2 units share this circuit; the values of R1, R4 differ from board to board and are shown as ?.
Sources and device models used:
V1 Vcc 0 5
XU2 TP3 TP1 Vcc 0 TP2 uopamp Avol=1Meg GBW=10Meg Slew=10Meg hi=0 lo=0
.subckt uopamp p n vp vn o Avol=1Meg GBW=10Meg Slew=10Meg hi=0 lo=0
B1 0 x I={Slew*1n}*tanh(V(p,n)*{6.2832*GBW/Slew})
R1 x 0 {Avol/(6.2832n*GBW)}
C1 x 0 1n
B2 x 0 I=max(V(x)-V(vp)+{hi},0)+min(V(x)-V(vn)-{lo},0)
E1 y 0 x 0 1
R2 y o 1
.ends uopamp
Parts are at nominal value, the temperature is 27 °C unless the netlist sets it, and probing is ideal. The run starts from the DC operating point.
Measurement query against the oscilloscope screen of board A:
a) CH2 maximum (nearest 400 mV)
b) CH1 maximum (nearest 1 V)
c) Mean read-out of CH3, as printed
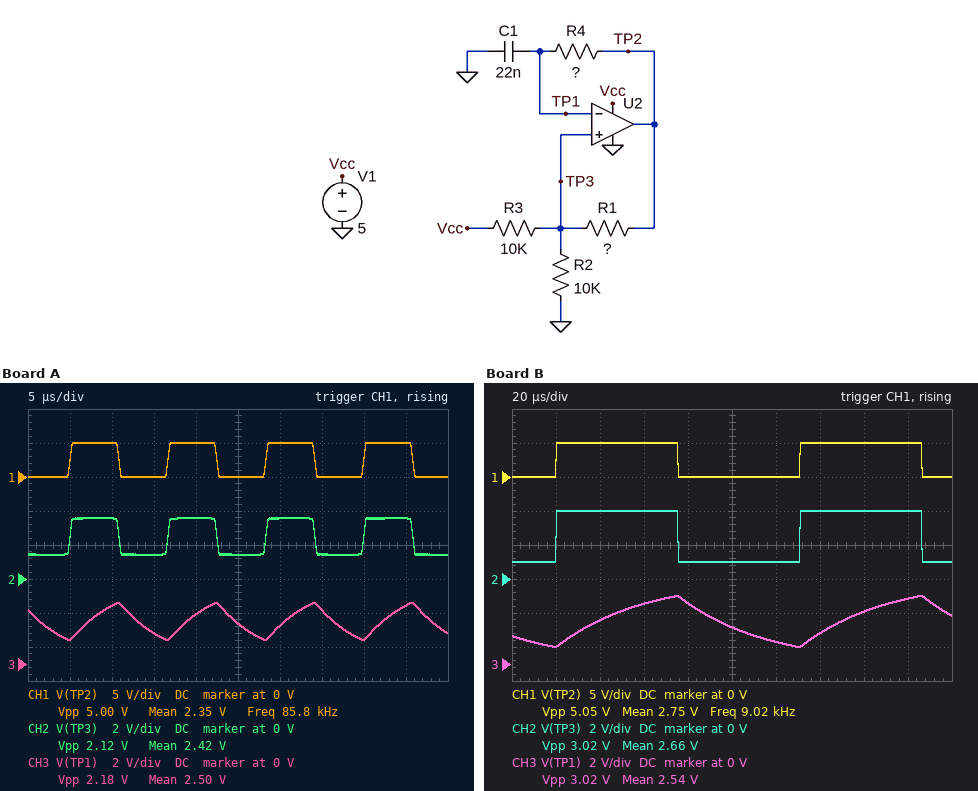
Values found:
3.6 V
5 V
2.50 V
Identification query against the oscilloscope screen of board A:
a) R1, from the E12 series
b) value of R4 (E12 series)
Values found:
6.8 kΩ
270 Ω
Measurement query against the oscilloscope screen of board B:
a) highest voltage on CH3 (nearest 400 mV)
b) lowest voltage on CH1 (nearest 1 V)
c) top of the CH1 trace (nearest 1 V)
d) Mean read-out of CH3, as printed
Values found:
4.0 V
0 V
5 V
2.54 V
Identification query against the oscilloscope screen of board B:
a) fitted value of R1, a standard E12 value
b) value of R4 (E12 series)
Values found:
3.3 kΩ
1.8 kΩ
